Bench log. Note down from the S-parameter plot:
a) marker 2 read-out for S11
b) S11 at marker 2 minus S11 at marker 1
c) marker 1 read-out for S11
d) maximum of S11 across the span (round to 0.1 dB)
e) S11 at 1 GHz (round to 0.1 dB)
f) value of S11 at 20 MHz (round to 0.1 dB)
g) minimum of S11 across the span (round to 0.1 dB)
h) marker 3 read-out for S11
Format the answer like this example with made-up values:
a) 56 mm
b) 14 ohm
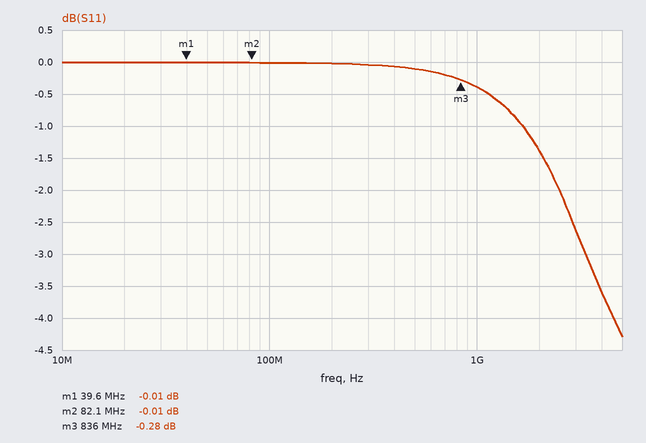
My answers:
a) -0.01 dB
b) 0.00 dB
c) -0.01 dB
d) 0.0 dB
e) -0.4 dB
f) 0.0 dB
g) -4.3 dB
h) -0.28 dB
